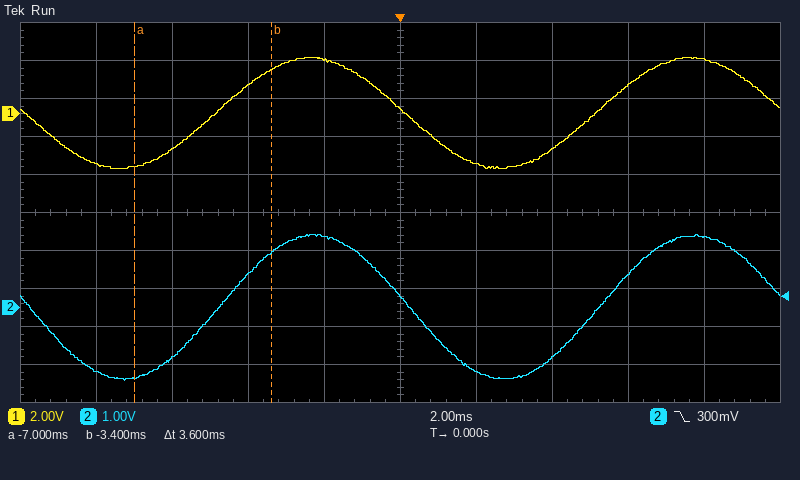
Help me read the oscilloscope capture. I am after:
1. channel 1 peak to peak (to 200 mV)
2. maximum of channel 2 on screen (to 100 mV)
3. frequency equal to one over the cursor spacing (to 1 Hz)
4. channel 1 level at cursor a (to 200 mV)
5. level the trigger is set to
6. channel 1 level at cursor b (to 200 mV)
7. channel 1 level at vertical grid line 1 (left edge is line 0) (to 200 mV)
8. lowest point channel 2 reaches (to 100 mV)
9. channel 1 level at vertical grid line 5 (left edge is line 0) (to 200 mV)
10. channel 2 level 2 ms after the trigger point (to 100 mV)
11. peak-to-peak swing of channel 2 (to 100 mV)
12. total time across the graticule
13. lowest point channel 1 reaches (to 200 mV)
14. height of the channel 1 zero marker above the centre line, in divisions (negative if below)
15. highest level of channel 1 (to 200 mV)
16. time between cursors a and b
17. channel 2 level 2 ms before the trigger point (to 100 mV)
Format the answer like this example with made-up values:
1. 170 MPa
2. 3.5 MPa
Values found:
1. 5.8 V
2. 1.9 V
3. 278 Hz
4. -2.8 V
5. 300 mV
6. 2.4 V
7. -2.6 V
8. -1.9 V
9. 200 mV
10. -1.7 V
11. 3.8 V
12. 20 ms
13. -2.8 V
14. +2.6 div
15. 3.0 V
16. 3.6 ms
17. 1.9 V
